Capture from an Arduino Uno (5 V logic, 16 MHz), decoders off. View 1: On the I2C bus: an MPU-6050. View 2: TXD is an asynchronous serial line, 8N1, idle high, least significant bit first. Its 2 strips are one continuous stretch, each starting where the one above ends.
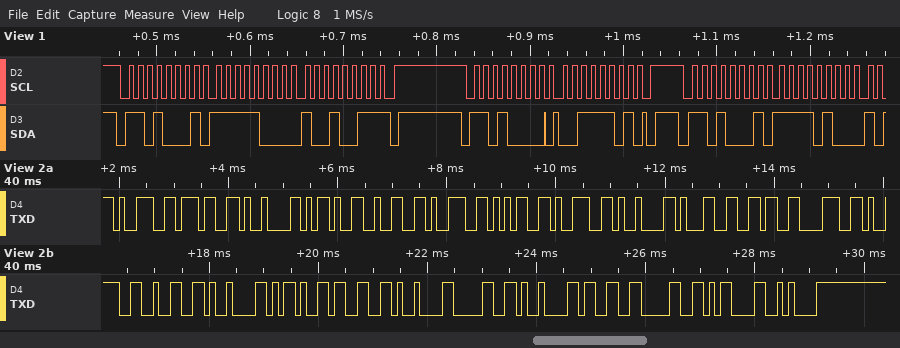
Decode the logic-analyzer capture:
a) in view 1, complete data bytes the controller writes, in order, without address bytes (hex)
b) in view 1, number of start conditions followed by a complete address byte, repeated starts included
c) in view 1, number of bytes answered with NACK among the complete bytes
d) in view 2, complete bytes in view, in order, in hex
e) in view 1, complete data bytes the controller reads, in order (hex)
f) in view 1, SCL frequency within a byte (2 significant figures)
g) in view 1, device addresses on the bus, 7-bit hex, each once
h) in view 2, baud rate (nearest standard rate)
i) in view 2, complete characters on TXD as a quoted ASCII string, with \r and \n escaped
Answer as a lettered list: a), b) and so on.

a) 3D
b) 3
c) 1
d) 39 37 09 2D 32 39 35 39 09 31 36 38 39 32 09 2D 33 09 30 09 33 30 0D 0A
e) F8 93 F4
f) 100 kHz
g) 0x68
h) 9600 baud
i) "97\t-2959\t16892\t-3\t0\t30\r\n"
